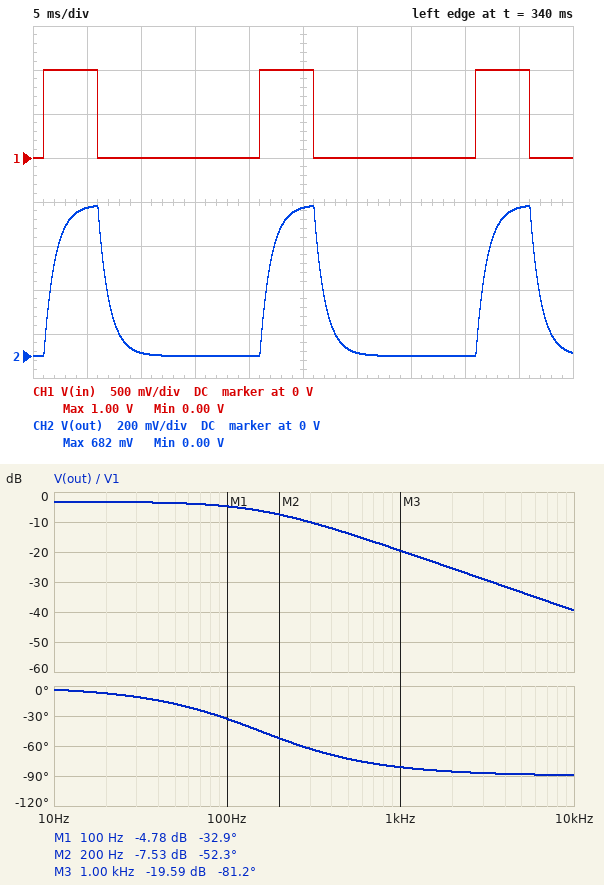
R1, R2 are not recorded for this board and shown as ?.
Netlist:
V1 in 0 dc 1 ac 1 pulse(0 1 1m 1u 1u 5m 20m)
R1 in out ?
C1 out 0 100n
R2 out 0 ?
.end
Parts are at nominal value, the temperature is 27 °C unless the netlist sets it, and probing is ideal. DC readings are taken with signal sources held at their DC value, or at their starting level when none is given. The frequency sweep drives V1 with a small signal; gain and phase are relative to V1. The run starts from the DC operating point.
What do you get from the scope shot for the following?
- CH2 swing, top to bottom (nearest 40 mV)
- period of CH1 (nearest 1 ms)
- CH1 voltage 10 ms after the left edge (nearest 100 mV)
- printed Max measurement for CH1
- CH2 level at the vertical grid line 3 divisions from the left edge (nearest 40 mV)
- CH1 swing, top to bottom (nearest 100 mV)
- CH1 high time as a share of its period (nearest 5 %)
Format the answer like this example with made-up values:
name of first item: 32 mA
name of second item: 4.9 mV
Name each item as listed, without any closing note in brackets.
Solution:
CH2 swing, top to bottom: 680 mV
period of CH1: 20 ms
CH1 voltage 10 ms after the left edge: 0 V
printed Max measurement for CH1: 1.00 V
CH2 level at the vertical grid line 3 divisions from the left edge: 0 V
CH1 swing, top to bottom: 1.0 V
CH1 high time as a share of its period: 25 %
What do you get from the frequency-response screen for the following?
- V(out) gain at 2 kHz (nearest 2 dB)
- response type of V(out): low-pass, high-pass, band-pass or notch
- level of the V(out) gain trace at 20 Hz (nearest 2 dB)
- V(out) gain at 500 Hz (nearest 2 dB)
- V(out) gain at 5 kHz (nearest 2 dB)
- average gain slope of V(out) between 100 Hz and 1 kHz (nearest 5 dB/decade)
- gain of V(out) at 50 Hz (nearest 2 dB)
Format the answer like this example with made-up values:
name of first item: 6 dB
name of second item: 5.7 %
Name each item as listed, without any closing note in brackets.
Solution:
V(out) gain at 2 kHz: -26 dB
response type of V(out): low-pass, high-pass, band-pass or notch: low-pass
level of the V(out) gain trace at 20 Hz: -4 dB
V(out) gain at 500 Hz: -14 dB
V(out) gain at 5 kHz: -34 dB
average gain slope of V(out) between 100 Hz and 1 kHz: -15 dB/decade
gain of V(out) at 50 Hz: -4 dB
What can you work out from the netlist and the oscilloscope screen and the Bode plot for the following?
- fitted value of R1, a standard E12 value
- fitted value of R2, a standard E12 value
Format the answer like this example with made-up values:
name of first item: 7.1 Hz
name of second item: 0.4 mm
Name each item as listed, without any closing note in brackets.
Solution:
fitted value of R1, a standard E12 value: 15 kΩ
fitted value of R2, a standard E12 value: 33 kΩ
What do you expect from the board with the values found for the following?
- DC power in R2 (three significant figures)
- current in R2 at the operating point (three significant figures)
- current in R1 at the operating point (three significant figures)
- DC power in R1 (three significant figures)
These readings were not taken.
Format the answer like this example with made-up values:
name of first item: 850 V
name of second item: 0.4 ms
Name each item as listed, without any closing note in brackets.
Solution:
DC power in R2: 14.3 µW
current in R2 at the operating point: 20.8 µA
current in R1 at the operating point: 20.8 µA
DC power in R1: 6.51 µW
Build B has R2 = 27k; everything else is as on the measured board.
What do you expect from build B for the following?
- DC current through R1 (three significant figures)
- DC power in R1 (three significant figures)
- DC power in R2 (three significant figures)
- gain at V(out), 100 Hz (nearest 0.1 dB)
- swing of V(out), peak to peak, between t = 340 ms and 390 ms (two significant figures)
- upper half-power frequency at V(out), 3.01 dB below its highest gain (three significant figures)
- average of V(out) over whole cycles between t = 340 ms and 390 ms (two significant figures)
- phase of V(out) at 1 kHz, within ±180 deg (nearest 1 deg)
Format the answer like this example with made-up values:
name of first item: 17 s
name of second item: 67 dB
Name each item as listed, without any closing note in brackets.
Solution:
DC current through R1: 23.8 µA
DC power in R1: 8.50 µW
DC power in R2: 15.3 µW
gain at V(out), 100 Hz: -5.2 dB
swing of V(out), peak to peak, between t = 340 ms and 390 ms: 640 mV
upper half-power frequency at V(out), 3.01 dB below its highest gain: 165 Hz
average of V(out) over whole cycles between t = 340 ms and 390 ms: 160 mV
phase of V(out) at 1 kHz, within ±180 deg: -81 deg
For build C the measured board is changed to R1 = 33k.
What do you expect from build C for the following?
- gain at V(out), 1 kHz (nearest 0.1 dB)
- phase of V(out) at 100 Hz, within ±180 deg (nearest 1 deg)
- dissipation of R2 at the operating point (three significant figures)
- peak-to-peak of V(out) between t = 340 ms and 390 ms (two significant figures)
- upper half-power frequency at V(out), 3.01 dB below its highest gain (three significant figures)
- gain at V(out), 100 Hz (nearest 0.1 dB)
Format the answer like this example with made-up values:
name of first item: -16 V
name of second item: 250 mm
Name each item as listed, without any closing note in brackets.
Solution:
gain at V(out), 1 kHz: -26.4 dB
phase of V(out) at 100 Hz, within ±180 deg: -46 deg
dissipation of R2 at the operating point: 7.58 µW
peak-to-peak of V(out) between t = 340 ms and 390 ms: 480 mV
upper half-power frequency at V(out), 3.01 dB below its highest gain: 96.5 Hz
gain at V(out), 100 Hz: -9.2 dB
